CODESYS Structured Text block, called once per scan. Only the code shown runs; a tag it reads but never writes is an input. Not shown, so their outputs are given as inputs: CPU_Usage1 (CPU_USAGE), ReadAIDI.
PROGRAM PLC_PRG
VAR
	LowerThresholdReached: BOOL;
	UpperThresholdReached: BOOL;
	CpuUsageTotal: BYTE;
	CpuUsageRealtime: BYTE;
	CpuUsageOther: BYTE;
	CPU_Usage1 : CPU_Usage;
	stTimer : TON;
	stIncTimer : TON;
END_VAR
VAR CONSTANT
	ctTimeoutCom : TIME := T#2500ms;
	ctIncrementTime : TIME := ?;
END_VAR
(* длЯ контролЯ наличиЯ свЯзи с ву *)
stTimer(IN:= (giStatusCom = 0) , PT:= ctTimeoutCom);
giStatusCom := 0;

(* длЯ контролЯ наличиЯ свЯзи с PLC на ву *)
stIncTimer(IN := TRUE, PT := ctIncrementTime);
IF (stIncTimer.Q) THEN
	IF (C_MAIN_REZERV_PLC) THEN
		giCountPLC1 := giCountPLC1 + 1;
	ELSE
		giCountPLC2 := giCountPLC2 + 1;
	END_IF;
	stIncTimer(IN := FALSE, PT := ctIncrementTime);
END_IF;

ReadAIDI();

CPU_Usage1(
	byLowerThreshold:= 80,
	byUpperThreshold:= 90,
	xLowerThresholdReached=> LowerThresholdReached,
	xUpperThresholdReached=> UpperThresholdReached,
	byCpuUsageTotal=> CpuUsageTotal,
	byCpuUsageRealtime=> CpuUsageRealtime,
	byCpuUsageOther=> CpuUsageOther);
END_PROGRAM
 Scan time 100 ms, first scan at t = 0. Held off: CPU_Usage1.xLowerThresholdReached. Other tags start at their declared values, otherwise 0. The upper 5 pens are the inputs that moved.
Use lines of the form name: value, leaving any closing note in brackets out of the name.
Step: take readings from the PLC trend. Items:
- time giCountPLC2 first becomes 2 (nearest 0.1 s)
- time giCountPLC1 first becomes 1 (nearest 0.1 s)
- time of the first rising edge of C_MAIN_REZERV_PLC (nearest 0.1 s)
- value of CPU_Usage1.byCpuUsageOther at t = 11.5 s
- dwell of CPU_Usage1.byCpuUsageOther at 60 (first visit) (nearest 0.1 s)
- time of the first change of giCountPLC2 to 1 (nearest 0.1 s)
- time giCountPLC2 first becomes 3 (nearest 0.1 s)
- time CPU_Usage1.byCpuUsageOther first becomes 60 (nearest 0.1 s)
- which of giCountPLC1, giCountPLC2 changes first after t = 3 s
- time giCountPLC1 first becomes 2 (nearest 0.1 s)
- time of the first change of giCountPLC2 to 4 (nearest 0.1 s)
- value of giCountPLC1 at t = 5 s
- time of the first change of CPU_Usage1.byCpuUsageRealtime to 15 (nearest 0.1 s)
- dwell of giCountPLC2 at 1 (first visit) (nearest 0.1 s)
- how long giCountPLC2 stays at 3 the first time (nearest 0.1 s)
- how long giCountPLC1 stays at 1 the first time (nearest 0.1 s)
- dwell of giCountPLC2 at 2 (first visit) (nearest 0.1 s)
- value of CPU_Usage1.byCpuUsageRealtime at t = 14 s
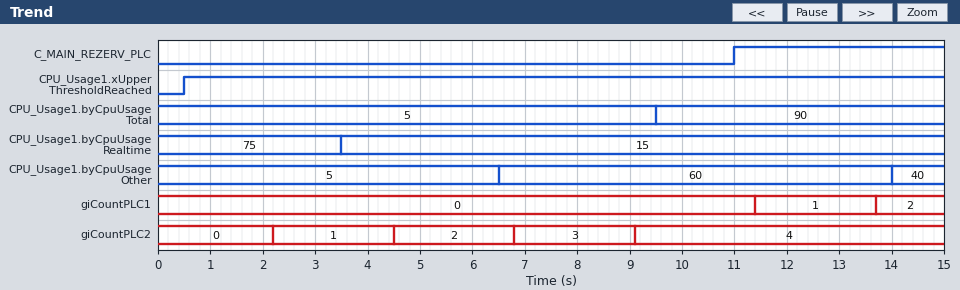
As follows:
time giCountPLC2 first becomes 2: 4.5 s
time giCountPLC1 first becomes 1: 11.4 s
time of the first rising edge of C_MAIN_REZERV_PLC: 11.0 s
value of CPU_Usage1.byCpuUsageOther at t = 11.5 s: 60
dwell of CPU_Usage1.byCpuUsageOther at 60 (first visit): 7.5 s
time of the first change of giCountPLC2 to 1: 2.2 s
time giCountPLC2 first becomes 3: 6.8 s
time CPU_Usage1.byCpuUsageOther first becomes 60: 6.5 s
which of giCountPLC1, giCountPLC2 changes first after t = 3 s: giCountPLC2
time giCountPLC1 first becomes 2: 13.7 s
time of the first change of giCountPLC2 to 4: 9.1 s
value of giCountPLC1 at t = 5 s: 0
time of the first change of CPU_Usage1.byCpuUsageRealtime to 15: 3.5 s
dwell of giCountPLC2 at 1 (first visit): 2.3 s
how long giCountPLC2 stays at 3 the first time: 2.3 s
how long giCountPLC1 stays at 1 the first time: 2.3 s
dwell of giCountPLC2 at 2 (first visit): 2.3 s
value of CPU_Usage1.byCpuUsageRealtime at t = 14 s: 15
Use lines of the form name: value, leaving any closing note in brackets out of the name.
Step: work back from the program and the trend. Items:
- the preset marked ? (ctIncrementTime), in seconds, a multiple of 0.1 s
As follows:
the preset marked ? (ctIncrementTime), in seconds, a multiple of 0.1 s: 2.2 s
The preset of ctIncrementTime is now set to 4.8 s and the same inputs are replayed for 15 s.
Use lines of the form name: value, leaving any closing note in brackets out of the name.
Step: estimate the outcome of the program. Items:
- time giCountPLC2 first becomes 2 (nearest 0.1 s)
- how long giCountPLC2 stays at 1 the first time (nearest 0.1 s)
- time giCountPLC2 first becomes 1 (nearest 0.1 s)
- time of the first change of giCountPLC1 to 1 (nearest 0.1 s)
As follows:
time giCountPLC2 first becomes 2: 9.7 s
how long giCountPLC2 stays at 1 the first time: 4.9 s
time giCountPLC2 first becomes 1: 4.8 s
time of the first change of giCountPLC1 to 1: 14.6 s
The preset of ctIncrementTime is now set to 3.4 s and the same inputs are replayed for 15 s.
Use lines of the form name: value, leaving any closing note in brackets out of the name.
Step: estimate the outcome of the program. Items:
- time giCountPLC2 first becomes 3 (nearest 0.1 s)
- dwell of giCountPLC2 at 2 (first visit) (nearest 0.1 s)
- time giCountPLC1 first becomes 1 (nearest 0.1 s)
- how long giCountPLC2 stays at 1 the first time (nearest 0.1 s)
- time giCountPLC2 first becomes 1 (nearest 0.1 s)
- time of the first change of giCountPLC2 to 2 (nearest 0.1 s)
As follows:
time giCountPLC2 first becomes 3: 10.4 s
dwell of giCountPLC2 at 2 (first visit): 3.5 s
time giCountPLC1 first becomes 1: 13.9 s
how long giCountPLC2 stays at 1 the first time: 3.5 s
time giCountPLC2 first becomes 1: 3.4 s
time of the first change of giCountPLC2 to 2: 6.9 s
